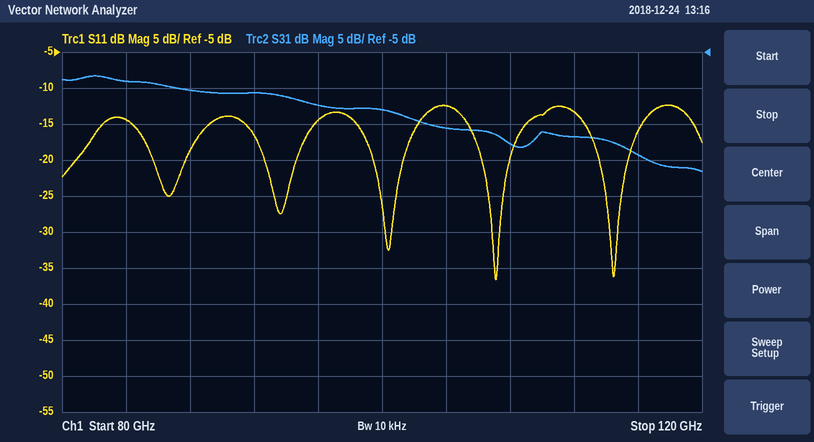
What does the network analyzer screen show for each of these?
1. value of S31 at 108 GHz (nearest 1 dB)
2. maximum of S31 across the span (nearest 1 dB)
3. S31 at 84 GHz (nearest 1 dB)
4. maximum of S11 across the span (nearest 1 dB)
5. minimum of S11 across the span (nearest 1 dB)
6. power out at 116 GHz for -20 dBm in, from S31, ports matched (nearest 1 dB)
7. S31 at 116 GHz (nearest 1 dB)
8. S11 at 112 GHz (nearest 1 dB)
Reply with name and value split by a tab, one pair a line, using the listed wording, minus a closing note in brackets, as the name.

value of S31 at 108 GHz	-18 dB
maximum of S31 across the span	-8 dB
S31 at 84 GHz	-9 dB
maximum of S11 across the span	-12 dB
minimum of S11 across the span	-37 dB
power out at 116 GHz for -20 dBm in, from S31, ports matched	-39 dBm
S31 at 116 GHz	-19 dB
S11 at 112 GHz	-13 dB
